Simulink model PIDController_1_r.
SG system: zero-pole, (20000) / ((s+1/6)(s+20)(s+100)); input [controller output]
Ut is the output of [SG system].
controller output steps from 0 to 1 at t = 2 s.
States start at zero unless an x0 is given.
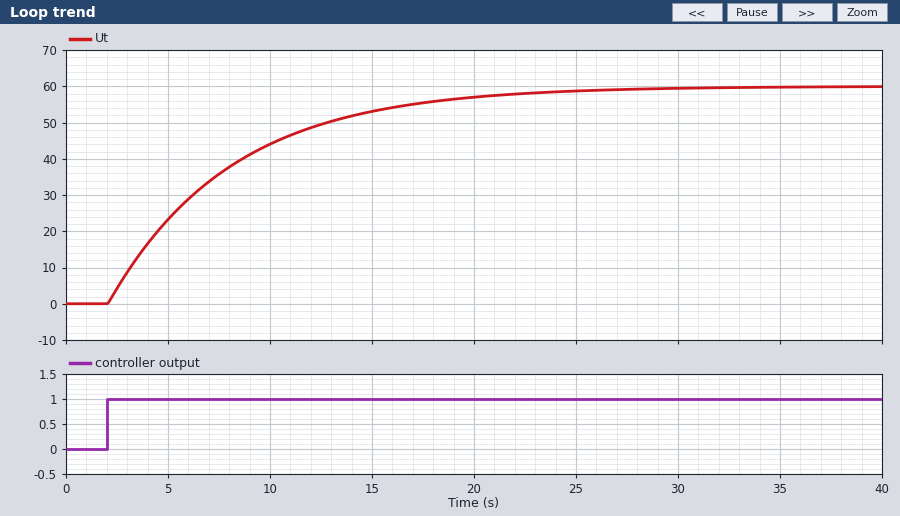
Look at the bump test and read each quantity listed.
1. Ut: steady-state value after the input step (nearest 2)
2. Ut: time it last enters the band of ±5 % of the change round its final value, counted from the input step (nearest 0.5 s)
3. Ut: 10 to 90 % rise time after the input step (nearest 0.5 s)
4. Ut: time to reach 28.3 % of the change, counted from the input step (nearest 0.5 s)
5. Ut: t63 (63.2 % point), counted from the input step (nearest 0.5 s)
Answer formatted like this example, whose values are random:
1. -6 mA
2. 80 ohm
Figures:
1. 60
2. 18.0 s
3. 13.0 s
4. 2.0 s
5. 6.0 s
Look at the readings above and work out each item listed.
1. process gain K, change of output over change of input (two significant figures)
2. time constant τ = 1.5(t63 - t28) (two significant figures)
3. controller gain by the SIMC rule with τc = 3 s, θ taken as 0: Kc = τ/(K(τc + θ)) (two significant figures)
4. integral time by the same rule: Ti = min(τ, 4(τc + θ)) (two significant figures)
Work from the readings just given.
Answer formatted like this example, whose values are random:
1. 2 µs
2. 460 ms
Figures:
1. 60
2. 6.0 s
3. 0.033
4. 6.0 s
